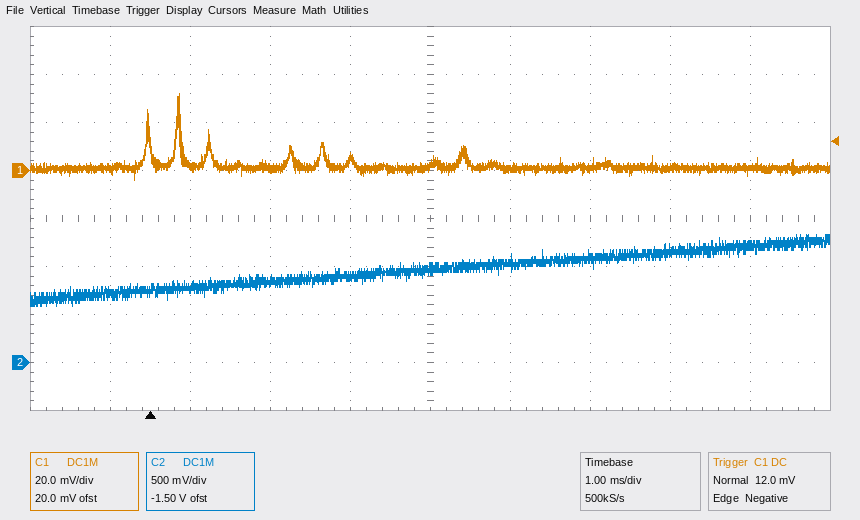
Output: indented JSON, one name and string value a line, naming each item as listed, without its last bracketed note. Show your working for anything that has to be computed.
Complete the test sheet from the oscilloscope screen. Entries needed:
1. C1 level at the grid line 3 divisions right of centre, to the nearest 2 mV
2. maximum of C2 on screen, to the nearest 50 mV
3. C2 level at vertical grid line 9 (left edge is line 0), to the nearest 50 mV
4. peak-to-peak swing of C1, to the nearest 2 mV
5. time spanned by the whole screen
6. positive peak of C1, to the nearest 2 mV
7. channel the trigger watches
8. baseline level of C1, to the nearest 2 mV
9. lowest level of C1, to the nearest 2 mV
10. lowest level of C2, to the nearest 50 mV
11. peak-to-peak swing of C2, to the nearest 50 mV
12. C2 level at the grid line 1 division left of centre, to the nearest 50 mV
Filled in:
{
  "C1 level at the grid line 3 divisions right of centre, to the nearest 2 mV": "2 mV",
  "maximum of C2 on screen, to the nearest 50 mV": "1.35 V",
  "C2 level at vertical grid line 9 (left edge is line 0), to the nearest 50 mV": "1.20 V",
  "peak-to-peak swing of C1, to the nearest 2 mV": "32 mV − (-4 mV) = 36 mV",
  "time spanned by the whole screen": "10 ms",
  "positive peak of C1, to the nearest 2 mV": "32 mV",
  "channel the trigger watches": "C1",
  "baseline level of C1, to the nearest 2 mV": "2 mV",
  "lowest level of C1, to the nearest 2 mV": "-4 mV",
  "lowest level of C2, to the nearest 50 mV": "600 mV",
  "peak-to-peak swing of C2, to the nearest 50 mV": "1.35 V − (600 mV) = 750 mV",
  "C2 level at the grid line 1 division left of centre, to the nearest 50 mV": "900 mV"
}
